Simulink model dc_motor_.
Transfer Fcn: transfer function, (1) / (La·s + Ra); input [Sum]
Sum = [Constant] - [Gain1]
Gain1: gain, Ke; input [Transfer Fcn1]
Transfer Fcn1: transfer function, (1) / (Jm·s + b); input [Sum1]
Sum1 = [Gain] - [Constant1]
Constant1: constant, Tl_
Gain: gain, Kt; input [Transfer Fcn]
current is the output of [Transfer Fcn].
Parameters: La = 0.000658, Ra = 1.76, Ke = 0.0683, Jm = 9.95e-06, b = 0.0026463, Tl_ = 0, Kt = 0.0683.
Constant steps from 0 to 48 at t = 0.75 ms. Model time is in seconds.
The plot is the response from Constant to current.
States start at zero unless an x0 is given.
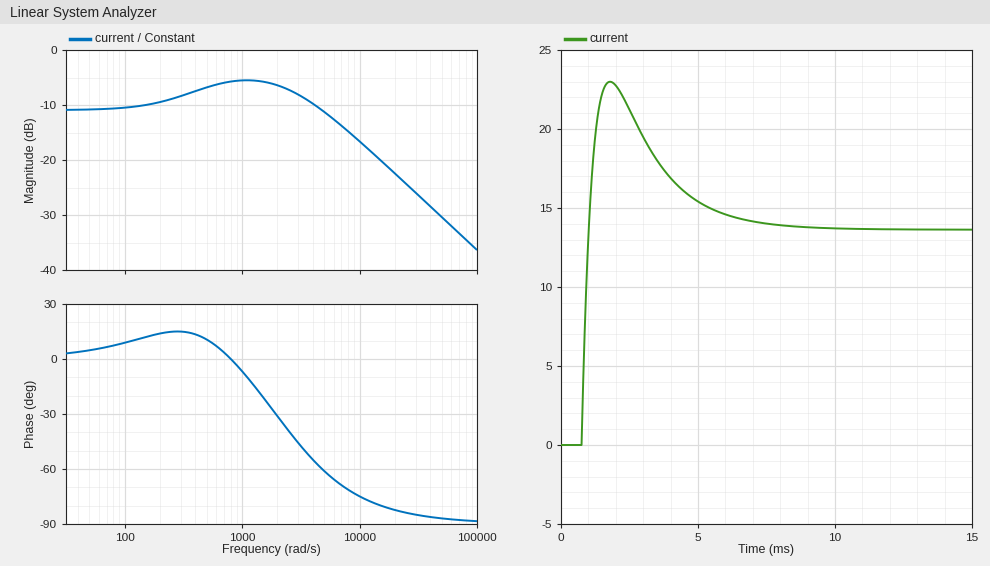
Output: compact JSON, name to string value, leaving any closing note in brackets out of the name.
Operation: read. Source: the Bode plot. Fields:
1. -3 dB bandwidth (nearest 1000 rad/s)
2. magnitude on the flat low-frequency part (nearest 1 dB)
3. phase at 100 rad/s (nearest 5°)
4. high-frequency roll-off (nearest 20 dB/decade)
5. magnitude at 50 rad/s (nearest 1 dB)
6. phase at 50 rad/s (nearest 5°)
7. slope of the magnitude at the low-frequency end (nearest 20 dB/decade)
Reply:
{"-3 dB bandwidth": "7000 rad/s", "magnitude on the flat low-frequency part": "-11 dB", "phase at 100 rad/s": "10°", "high-frequency roll-off": "-20 dB/decade", "magnitude at 50 rad/s": "-11 dB", "phase at 50 rad/s": "5°", "slope of the magnitude at the low-frequency end": "0 dB/decade"}
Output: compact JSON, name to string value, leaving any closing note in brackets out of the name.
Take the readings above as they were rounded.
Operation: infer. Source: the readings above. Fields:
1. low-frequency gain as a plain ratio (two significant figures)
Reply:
{"low-frequency gain as a plain ratio": "0.28"}
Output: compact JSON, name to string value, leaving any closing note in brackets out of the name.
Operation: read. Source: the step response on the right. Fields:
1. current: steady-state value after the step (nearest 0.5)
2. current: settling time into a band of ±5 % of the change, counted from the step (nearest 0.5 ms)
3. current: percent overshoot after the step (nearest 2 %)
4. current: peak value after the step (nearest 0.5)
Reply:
{"current: steady-state value after the step": "13.5", "current: settling time into a band of ±5 % of the change, counted from the step": "6.0 ms", "current: percent overshoot after the step": "68 %", "current: peak value after the step": "23.0"}
